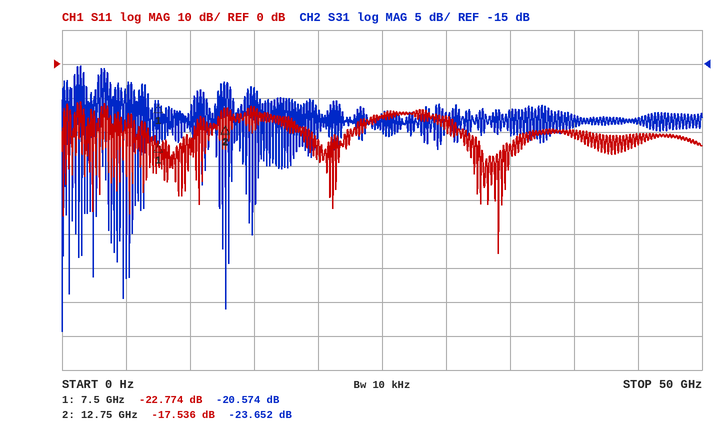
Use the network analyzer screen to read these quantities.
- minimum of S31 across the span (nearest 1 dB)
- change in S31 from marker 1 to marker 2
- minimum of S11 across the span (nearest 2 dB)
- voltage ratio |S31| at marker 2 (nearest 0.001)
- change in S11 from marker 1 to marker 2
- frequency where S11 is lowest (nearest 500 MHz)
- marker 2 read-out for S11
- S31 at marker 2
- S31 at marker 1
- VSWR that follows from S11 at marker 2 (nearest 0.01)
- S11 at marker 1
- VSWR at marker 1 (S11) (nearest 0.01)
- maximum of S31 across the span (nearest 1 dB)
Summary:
-54 dB
-3.078 dB
-56 dB
0.066
5.238 dB
34.0 GHz
-17.536 dB
-23.652 dB
-20.574 dB
1.31
-22.774 dB
1.16
-15 dB
